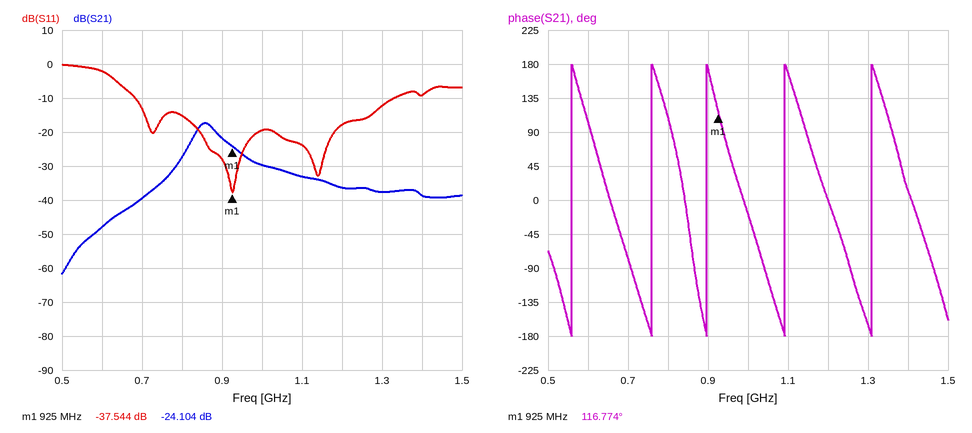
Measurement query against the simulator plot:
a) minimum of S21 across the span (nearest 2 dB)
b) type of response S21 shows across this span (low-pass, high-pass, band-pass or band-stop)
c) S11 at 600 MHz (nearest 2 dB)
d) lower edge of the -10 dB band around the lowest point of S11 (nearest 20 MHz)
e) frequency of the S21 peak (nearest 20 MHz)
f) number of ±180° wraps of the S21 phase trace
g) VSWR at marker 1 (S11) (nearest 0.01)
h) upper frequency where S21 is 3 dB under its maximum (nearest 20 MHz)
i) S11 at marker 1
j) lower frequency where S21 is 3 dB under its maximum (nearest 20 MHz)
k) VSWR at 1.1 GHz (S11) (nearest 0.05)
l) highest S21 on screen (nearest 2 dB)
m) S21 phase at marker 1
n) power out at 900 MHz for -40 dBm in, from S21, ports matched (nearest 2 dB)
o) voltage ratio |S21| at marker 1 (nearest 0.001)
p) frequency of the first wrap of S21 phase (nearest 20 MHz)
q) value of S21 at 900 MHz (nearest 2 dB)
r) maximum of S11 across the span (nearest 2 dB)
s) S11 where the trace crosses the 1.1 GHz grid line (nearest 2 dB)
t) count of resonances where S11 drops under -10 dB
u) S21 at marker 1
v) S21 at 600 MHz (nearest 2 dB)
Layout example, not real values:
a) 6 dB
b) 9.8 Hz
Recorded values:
a) -62 dB
b) band-pass
c) -2 dB
d) 680 MHz
e) 860 MHz
f) 5
g) 1.03
h) 880 MHz
i) -37.544 dB
j) 840 MHz
k) 1.15
l) -18 dB
m) 116.774°
n) -62 dBm
o) 0.062
p) 560 MHz
q) -22 dB
r) 0 dB
s) -24 dB
t) 3
u) -24.104 dB
v) -48 dB
